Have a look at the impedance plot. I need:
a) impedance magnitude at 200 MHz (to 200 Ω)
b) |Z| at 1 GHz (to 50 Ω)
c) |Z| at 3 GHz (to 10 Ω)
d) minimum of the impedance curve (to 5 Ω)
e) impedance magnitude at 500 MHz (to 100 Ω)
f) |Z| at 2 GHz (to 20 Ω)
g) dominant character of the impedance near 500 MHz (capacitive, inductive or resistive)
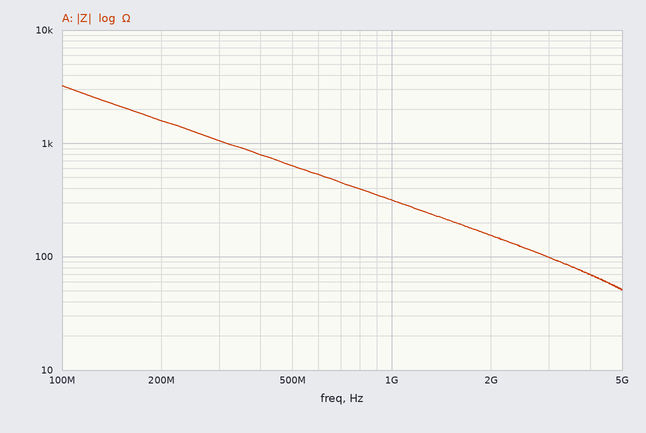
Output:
1.6 kΩ
300 Ω
100 Ω
50 Ω
600 Ω
160 Ω
capacitive
